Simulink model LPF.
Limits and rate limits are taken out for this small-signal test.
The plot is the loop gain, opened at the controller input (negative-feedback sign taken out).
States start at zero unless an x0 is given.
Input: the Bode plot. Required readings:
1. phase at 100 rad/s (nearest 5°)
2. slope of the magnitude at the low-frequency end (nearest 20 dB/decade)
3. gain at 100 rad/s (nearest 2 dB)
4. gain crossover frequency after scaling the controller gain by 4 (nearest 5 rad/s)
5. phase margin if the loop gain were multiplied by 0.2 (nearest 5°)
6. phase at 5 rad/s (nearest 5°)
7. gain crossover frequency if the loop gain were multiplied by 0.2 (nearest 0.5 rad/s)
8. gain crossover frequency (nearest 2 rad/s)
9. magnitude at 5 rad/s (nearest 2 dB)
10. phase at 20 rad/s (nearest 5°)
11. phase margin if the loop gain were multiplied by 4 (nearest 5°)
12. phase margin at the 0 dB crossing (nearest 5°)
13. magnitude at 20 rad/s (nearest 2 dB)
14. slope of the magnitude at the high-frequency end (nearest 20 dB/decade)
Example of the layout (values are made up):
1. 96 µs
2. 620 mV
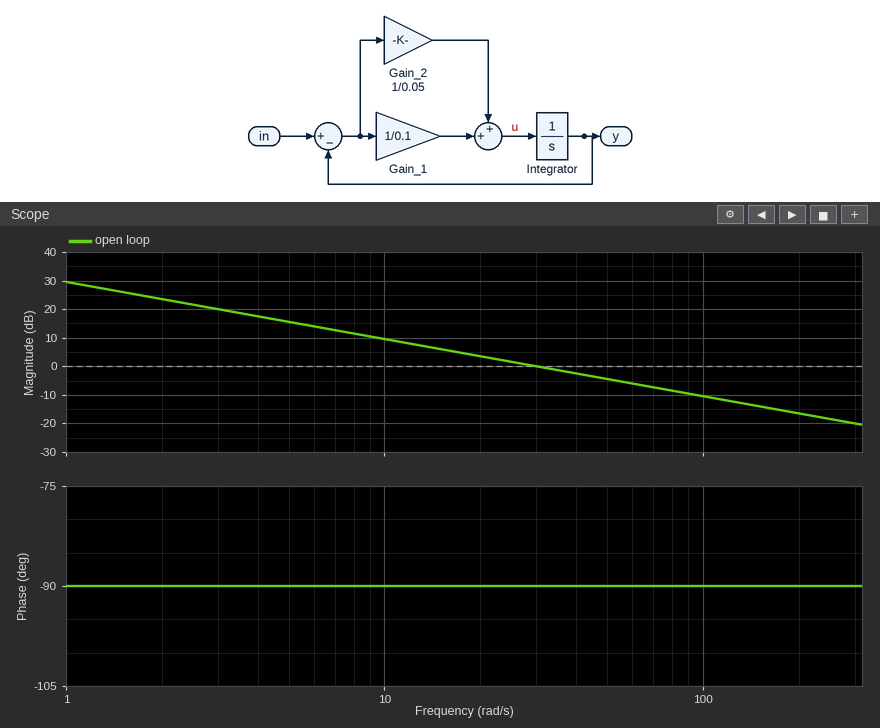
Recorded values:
1. -90°
2. -20 dB/decade
3. -10 dB
4. 120 rad/s
5. 90°
6. -90°
7. 6.0 rad/s
8. 30 rad/s
9. 16 dB
10. -90°
11. 90°
12. 90°
13. 4 dB
14. -20 dB/decade
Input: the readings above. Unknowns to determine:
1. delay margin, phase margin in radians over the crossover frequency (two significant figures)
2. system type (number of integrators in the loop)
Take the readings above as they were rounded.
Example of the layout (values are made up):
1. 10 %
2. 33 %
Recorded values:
1. 0.052 s
2. 1
